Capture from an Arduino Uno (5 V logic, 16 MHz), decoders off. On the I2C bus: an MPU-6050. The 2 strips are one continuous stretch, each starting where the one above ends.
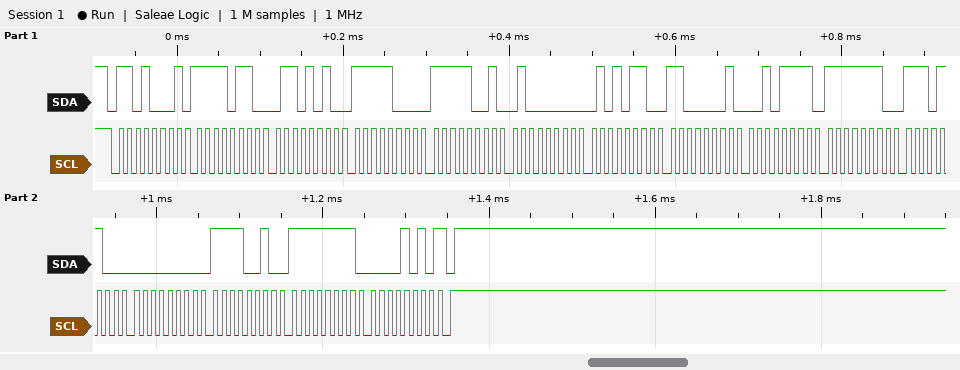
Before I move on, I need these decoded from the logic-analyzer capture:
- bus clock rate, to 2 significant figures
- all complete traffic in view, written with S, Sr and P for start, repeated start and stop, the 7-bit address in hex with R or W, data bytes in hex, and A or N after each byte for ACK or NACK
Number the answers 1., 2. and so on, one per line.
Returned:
1. 100 kHz
2. S 68R A F6 A 6A A F8 A F9 A 40 A 56 A C1 A 2F A FE A EC A 00 A F2 A FF A 0A N P
